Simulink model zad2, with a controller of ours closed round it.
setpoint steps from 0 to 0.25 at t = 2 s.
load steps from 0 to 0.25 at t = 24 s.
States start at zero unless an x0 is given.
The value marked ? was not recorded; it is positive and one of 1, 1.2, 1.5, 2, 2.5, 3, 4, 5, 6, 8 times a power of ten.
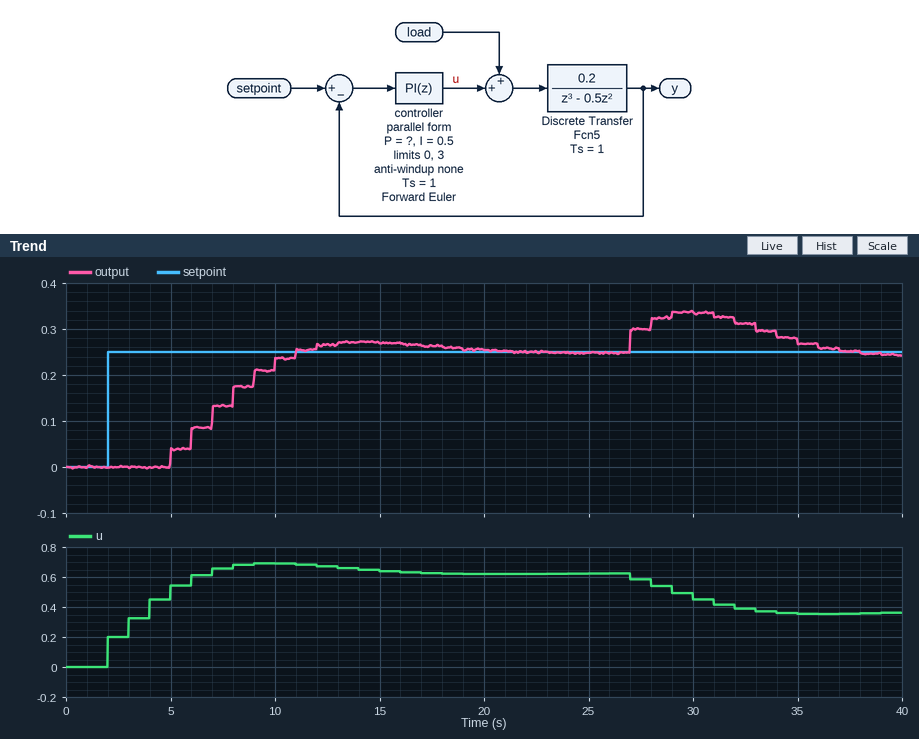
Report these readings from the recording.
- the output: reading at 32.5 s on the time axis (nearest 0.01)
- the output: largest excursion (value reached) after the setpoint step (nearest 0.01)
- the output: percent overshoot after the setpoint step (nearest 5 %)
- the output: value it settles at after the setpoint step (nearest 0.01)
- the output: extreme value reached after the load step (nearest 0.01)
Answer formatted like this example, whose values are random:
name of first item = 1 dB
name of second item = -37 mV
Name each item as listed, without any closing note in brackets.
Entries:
the output: reading at 32.5 s on the time axis = 0.31
the output: largest excursion (value reached) after the setpoint step = 0.27
the output: percent overshoot after the setpoint step = 10 %
the output: value it settles at after the setpoint step = 0.25
the output: extreme value reached after the load step = 0.34
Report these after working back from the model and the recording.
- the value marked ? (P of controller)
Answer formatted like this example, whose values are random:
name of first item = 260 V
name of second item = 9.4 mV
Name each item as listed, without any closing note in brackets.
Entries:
the value marked ? = 0.8
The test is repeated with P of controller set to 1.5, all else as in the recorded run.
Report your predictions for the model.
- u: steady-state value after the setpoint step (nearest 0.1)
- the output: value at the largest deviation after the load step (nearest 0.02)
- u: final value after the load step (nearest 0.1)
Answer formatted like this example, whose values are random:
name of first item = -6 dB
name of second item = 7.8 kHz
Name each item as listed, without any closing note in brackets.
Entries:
u: steady-state value after the setpoint step = 0.6
the output: value at the largest deviation after the load step = 0.34
u: final value after the load step = 0.4
